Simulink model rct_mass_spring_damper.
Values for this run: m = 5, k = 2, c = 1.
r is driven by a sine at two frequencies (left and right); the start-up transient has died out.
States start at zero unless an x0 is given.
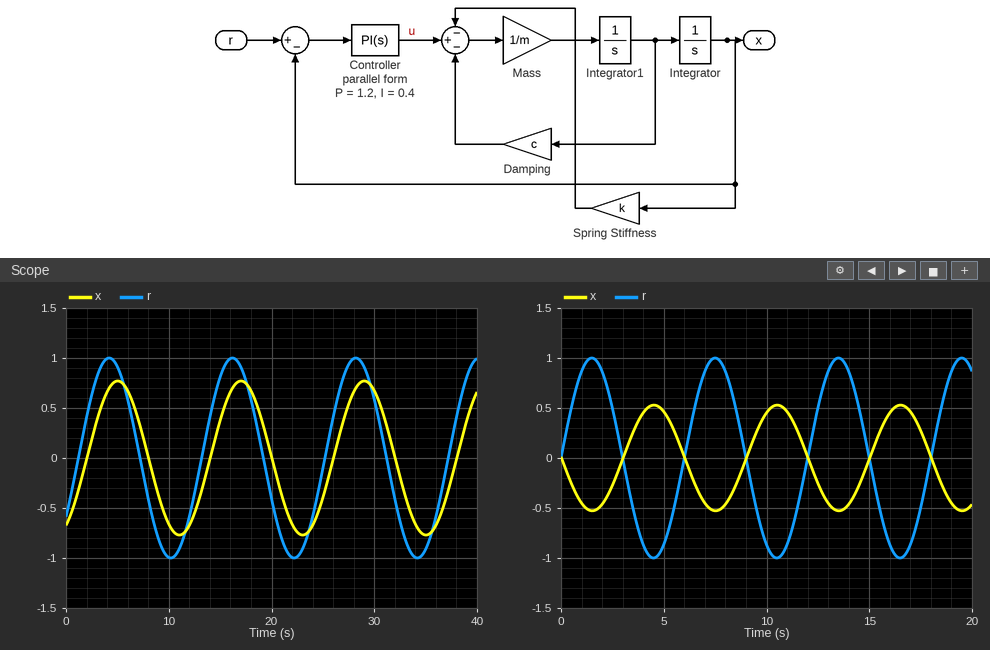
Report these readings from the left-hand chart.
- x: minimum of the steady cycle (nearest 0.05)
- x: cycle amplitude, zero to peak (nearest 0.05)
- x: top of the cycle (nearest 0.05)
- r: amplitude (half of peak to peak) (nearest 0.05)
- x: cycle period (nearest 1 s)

-0.75
0.75
0.75
1.00
12 s
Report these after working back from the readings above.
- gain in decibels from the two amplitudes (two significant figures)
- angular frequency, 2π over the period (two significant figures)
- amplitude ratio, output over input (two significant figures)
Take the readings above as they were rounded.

-2.5 dB
0.52 rad/s
0.75
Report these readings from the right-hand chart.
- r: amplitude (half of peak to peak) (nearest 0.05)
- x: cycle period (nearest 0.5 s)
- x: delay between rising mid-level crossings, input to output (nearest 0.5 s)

1.00
6.0 s
3.0 s
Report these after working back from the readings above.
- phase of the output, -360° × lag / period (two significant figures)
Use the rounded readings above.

-180°
